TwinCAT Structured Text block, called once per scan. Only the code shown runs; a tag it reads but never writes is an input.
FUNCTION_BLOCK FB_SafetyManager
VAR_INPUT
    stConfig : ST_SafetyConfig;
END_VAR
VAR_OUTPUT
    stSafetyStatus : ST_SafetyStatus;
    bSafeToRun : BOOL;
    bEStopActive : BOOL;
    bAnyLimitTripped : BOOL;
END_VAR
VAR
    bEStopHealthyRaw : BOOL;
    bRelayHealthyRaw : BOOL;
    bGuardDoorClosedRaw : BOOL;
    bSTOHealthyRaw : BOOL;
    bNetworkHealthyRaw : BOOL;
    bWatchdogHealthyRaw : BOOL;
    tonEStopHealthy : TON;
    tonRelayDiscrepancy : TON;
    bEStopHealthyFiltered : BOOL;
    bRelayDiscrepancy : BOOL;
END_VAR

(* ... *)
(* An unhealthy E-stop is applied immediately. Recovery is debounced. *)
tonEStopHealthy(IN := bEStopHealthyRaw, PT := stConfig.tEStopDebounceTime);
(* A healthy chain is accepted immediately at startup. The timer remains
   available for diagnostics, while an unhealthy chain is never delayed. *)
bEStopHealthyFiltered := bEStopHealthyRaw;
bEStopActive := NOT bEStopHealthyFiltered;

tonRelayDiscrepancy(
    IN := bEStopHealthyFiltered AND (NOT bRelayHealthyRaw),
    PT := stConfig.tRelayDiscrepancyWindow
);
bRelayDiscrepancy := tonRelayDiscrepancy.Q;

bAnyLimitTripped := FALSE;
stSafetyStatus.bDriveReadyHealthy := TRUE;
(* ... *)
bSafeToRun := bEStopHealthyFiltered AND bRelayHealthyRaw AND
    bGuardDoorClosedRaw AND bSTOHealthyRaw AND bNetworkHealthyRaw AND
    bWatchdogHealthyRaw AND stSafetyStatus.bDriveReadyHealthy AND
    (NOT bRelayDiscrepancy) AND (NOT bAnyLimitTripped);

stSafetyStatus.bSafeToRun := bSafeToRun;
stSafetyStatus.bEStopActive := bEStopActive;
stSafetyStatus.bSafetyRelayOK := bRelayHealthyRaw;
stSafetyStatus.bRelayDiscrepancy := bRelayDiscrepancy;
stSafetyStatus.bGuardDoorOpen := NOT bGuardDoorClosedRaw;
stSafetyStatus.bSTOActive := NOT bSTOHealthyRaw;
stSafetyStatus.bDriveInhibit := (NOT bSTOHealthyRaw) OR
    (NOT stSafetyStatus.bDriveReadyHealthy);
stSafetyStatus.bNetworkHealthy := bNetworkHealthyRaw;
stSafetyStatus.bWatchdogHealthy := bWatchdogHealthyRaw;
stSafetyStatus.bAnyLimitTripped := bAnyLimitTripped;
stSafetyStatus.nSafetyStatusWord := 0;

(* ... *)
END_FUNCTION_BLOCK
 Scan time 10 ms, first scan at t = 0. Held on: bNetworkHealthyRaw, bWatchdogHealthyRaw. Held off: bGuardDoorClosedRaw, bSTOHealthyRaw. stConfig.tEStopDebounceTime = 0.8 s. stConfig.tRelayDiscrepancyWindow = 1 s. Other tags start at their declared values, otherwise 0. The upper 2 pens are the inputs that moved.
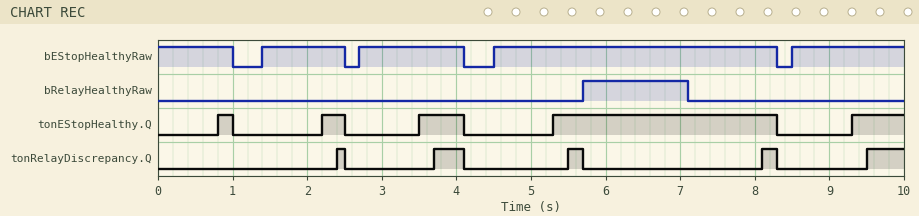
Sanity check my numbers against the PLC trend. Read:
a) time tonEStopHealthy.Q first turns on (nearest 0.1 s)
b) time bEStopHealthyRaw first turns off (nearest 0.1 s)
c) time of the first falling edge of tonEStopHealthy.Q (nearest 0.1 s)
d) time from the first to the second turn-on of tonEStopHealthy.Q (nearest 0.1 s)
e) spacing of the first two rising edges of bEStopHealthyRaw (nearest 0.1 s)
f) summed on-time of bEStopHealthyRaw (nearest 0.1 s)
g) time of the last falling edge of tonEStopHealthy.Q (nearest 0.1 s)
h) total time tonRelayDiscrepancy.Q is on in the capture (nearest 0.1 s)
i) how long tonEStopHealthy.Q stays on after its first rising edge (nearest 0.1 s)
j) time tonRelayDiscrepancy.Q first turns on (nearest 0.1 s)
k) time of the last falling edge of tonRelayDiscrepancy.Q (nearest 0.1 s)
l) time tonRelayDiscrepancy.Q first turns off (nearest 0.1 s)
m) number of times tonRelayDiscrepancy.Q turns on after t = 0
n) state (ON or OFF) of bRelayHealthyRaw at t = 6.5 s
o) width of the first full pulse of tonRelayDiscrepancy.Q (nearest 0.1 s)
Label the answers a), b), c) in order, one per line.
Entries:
a) 0.8 s
b) 1.0 s
c) 1.0 s
d) 1.4 s
e) 1.3 s
f) 8.8 s
g) 8.3 s
h) 1.4 s
i) 0.2 s
j) 2.4 s
k) 8.3 s
l) 2.5 s
m) 5
n) ON
o) 0.1 s
